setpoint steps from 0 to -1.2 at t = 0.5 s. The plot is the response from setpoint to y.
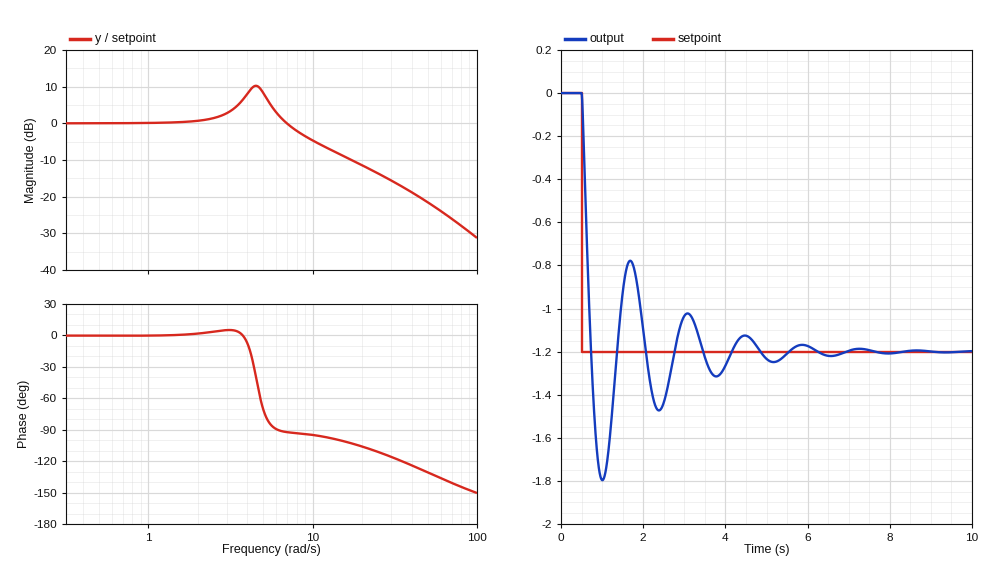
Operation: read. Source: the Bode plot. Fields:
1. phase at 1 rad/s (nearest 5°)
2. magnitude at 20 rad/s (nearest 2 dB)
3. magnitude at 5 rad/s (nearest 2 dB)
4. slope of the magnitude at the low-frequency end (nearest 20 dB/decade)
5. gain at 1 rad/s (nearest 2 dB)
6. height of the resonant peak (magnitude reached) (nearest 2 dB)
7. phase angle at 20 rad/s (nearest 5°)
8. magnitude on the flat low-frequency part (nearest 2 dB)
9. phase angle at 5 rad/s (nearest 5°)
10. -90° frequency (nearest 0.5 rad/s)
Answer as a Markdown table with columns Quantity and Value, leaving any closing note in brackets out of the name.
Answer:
| Quantity | Value |
|---|---|
| phase at 1 rad/s | 0° |
| magnitude at 20 rad/s | -12 dB |
| magnitude at 5 rad/s | 8 dB |
| slope of the magnitude at the low-frequency end | 0 dB/decade |
| gain at 1 rad/s | 0 dB |
| height of the resonant peak (magnitude reached) | 10 dB |
| phase angle at 20 rad/s | -105° |
| magnitude on the flat low-frequency part | 0 dB |
| phase angle at 5 rad/s | -70° |
| -90° frequency | 6.0 rad/s |
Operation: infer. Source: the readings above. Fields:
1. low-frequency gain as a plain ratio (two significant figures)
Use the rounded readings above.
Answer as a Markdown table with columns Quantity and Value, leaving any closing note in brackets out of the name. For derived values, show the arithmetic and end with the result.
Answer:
| Quantity | Value |
|---|---|
| low-frequency gain as a plain ratio | 10^(0 / 20) = 1.0 |
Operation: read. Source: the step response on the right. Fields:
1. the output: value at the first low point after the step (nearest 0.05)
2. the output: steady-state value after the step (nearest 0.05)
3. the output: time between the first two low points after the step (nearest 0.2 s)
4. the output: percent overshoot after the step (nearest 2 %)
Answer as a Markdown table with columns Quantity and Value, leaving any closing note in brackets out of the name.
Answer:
| Quantity | Value |
|---|---|
| the output: value at the first low point after the step | -1.80 |
| the output: steady-state value after the step | -1.20 |
| the output: time between the first two low points after the step | 1.4 s |
| the output: percent overshoot after the step | 50 % |
